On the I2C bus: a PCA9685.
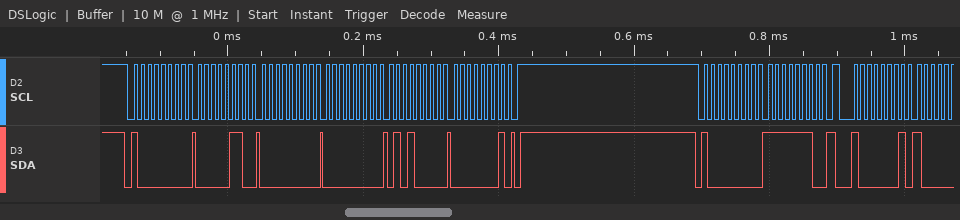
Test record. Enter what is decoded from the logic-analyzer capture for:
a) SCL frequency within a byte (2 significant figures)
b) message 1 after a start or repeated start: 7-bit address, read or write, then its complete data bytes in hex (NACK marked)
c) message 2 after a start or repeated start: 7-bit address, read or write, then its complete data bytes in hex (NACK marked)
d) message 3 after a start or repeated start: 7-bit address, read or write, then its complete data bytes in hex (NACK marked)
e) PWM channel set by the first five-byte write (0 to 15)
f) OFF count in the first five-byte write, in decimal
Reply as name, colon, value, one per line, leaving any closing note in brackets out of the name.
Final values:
SCL frequency within a byte: 100 kHz
message 1 after a start or repeated start: 7-bit address, read or write, then its complete data bytes in hex: 0x40 write: 06 00 00 50 01
message 2 after a start or repeated start: 7-bit address, read or write, then its complete data bytes in hex: 0x40 write: FE
message 3 after a start or repeated start: 7-bit address, read or write, then its complete data bytes in hex: 0x40 read
PWM channel set by the first five-byte write: 0
OFF count in the first five-byte write, in decimal: 336
